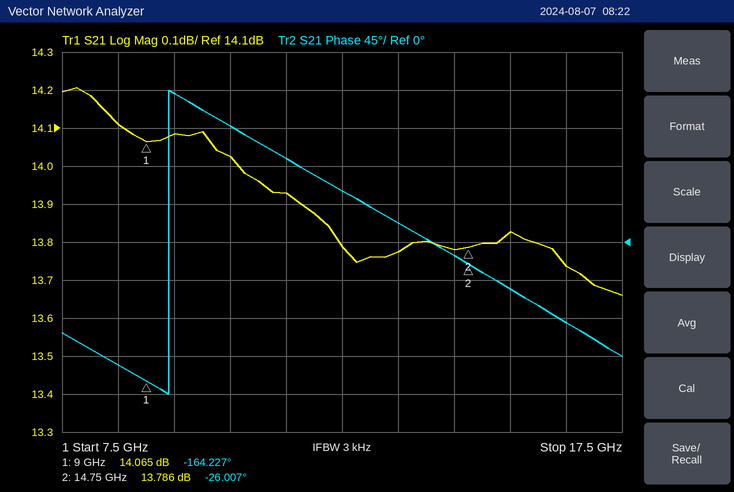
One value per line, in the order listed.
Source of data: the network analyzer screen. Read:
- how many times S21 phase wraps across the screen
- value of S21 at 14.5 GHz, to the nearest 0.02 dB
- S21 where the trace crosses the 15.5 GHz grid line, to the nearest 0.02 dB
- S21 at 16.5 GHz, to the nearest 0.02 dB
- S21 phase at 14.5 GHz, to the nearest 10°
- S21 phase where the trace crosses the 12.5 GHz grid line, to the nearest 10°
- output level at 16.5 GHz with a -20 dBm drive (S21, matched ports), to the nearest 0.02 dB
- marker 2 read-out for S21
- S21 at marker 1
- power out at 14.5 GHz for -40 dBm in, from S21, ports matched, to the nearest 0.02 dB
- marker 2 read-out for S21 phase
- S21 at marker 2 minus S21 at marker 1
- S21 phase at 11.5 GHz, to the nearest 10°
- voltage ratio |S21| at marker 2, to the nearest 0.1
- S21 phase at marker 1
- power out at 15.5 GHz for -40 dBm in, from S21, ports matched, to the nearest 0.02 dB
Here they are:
1
13.78 dB
13.82 dB
13.74 dB
-20°
60°
-6.26 dBm
13.786 dB
14.065 dB
-26.22 dBm
-26.007°
-0.279 dB
100°
4.9
-164.227°
-26.18 dBm
